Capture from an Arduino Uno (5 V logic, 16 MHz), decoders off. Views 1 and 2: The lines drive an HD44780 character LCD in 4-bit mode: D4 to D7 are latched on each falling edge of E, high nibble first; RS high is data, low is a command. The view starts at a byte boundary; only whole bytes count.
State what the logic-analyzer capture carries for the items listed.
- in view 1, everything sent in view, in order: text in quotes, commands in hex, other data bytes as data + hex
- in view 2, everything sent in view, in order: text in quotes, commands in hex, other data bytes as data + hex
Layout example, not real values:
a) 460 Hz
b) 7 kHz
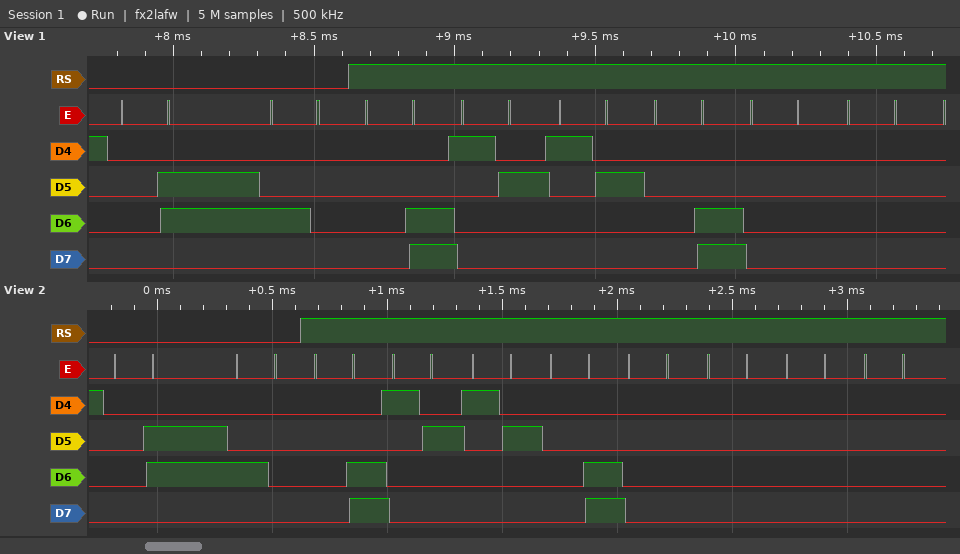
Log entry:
a) 0x06 0x40 data 0C 12 12 0C 00 00
b) 0x06 0x40 data 0C 12 12 0C 00 00 00 00
